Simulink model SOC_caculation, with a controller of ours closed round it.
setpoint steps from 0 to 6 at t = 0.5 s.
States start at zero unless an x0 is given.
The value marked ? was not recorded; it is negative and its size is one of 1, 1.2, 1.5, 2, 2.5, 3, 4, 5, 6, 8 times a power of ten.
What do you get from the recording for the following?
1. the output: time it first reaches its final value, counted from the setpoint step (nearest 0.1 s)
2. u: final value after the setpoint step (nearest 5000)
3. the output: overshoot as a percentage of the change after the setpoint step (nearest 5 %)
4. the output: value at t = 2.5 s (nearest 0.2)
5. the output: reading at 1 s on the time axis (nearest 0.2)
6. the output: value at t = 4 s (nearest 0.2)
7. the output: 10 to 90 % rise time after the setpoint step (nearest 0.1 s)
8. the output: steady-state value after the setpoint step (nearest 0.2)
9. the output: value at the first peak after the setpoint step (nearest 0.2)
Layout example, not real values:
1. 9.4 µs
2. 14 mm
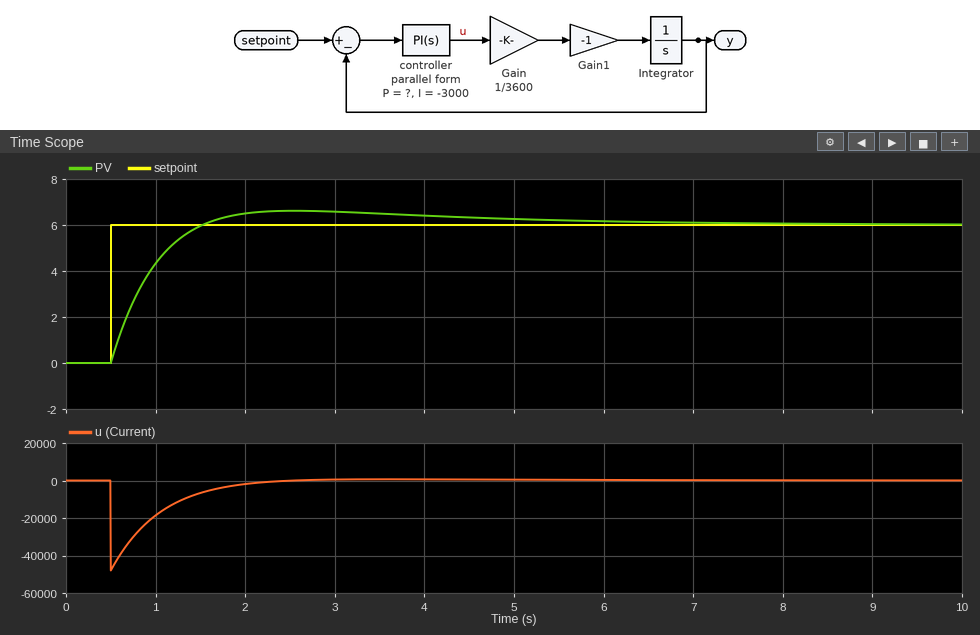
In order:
1. 1.0 s
2. 0
3. 10 %
4. 6.6
5. 4.4
6. 6.4
7. 0.7 s
8. 6.0
9. 6.6
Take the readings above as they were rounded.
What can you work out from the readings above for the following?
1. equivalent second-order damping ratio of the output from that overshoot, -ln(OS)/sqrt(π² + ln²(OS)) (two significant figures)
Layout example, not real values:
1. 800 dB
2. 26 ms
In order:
1. 0.59
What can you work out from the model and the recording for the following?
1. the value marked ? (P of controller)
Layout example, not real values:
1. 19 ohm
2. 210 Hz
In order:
1. -8000
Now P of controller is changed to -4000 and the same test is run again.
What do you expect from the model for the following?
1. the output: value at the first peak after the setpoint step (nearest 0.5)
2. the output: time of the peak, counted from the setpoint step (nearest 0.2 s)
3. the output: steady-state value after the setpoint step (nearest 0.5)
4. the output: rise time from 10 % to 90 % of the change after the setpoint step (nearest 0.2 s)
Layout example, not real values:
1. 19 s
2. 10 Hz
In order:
1. 7.5
2. 2.6 s
3. 6.0
4. 1.0 s
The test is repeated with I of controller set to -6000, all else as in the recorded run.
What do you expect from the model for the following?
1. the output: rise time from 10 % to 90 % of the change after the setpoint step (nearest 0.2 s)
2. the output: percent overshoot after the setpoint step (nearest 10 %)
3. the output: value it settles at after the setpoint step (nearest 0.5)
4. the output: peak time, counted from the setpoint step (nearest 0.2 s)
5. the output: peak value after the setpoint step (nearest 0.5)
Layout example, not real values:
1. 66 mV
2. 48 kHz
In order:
1. 0.6 s
2. 20 %
3. 6.0
4. 1.6 s
5. 7.0
